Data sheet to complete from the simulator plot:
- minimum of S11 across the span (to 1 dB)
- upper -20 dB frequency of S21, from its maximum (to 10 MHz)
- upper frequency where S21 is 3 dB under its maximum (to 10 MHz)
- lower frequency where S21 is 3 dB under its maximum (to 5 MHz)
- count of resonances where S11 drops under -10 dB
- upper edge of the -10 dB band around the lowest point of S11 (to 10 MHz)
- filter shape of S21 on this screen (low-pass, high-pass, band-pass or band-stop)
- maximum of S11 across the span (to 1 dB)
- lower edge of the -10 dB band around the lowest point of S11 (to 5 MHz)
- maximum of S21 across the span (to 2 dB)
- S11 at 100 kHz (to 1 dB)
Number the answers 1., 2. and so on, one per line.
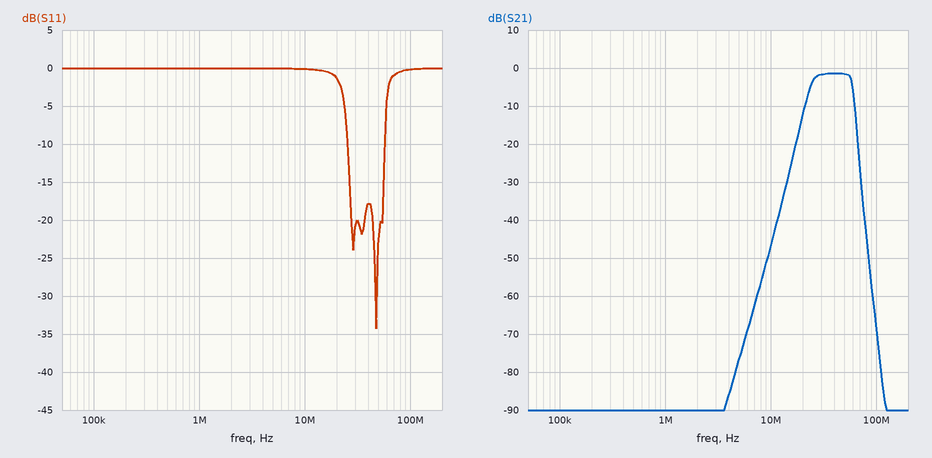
1. -34 dB
2. 70 MHz
3. 60 MHz
4. 25 MHz
5. 2
6. 60 MHz
7. band-pass
8. 0 dB
9. 25 MHz
10. -2 dB
11. 0 dB
